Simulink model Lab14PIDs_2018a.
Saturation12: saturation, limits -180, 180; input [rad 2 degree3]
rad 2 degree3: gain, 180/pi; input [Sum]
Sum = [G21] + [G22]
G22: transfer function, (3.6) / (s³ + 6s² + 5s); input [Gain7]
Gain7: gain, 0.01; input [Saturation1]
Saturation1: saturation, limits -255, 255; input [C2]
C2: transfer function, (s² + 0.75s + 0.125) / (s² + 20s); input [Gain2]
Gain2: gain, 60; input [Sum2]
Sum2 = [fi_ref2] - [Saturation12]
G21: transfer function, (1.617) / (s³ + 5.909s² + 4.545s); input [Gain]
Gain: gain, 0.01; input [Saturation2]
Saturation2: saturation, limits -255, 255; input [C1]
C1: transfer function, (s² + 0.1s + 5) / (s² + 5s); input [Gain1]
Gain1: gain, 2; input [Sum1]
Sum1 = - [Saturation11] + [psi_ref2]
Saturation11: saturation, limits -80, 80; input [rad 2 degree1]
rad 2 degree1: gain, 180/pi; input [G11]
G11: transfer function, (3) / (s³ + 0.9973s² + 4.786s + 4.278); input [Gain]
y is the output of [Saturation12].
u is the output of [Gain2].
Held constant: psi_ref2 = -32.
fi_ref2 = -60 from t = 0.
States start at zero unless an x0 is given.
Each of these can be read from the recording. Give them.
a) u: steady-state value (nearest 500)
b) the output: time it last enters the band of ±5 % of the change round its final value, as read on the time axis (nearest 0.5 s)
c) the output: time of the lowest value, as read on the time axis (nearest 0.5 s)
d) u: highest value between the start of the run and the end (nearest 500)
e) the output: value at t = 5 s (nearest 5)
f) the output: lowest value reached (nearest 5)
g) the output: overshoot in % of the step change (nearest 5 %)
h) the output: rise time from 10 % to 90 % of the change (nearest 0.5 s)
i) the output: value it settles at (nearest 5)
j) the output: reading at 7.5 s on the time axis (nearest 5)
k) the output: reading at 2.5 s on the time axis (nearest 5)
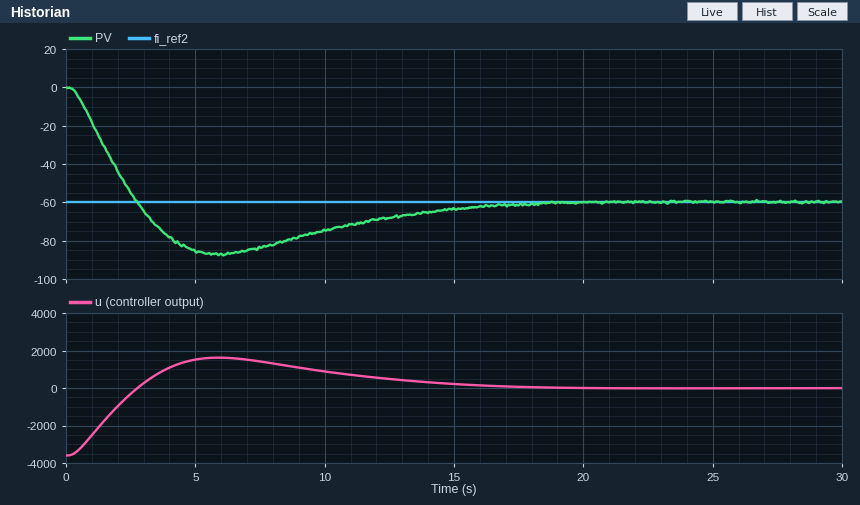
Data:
0
15.5 s
6.0 s
1500
-85
-85
45 %
2.0 s
-60
-85
-55
